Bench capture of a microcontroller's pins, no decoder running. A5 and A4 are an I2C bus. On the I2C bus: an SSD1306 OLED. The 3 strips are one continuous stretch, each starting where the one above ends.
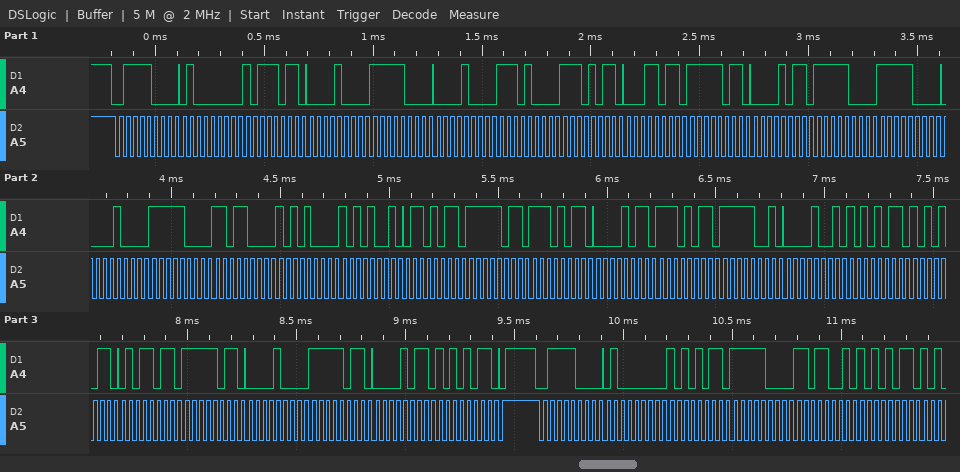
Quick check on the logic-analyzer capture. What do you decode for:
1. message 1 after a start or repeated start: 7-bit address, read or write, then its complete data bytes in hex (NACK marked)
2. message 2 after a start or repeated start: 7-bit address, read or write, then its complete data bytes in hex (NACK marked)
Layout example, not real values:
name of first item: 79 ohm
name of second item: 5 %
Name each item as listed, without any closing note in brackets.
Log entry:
message 1 after a start or repeated start: 7-bit address, read or write, then its complete data bytes in hex: 0x3C write: 40 BB 08 F8 08 E8 EB 1B FB 0B F8 F8 08 F8 D8 A8 A9 6B FB EB 0B EB F9 09 AB AB 5B FB 08 FB 0B AB
message 2 after a start or repeated start: 7-bit address, read or write, then its complete data bytes in hex: 0x3C write: 40 AB F8 D9 AB
